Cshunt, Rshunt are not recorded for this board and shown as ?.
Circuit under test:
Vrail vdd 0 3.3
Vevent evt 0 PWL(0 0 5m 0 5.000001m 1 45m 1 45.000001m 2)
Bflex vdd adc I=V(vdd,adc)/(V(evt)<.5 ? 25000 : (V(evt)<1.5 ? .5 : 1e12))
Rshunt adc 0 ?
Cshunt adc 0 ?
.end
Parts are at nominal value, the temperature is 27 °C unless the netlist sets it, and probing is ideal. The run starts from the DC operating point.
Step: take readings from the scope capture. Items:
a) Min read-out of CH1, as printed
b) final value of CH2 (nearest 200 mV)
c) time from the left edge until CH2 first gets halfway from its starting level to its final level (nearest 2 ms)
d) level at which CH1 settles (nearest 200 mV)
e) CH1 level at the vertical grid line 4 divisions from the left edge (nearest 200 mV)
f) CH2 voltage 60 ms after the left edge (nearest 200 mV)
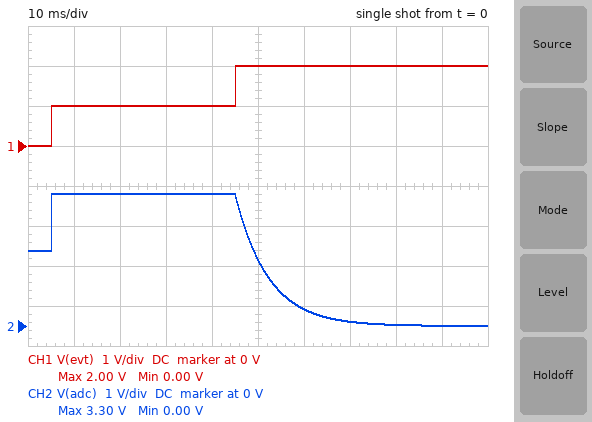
0.00 V
0 V
54 ms
2.0 V
1.0 V
400 mV
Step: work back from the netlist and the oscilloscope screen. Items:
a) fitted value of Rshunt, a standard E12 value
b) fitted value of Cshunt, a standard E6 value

33 kΩ
220 nF
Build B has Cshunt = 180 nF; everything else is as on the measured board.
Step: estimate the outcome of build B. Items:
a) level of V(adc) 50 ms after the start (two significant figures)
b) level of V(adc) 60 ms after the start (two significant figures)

1.4 V
260 mV
